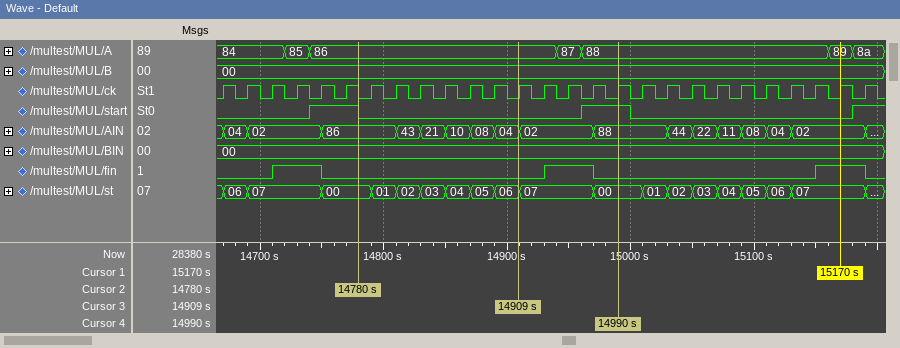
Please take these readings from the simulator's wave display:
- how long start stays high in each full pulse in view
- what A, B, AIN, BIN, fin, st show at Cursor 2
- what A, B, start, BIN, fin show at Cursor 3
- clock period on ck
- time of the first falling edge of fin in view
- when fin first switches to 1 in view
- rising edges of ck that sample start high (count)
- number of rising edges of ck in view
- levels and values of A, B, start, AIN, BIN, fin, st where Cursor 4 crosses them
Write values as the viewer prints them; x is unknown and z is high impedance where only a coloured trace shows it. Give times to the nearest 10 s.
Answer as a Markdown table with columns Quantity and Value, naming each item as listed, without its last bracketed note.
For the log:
| Quantity | Value |
|---|---|
| how long start stays high in each full pulse in view | 40 s, 40 s |
| what A, B, AIN, BIN, fin, st show at Cursor 2 | A=86, B=00, AIN=86, BIN=00, fin=0, st=00 |
| what A, B, start, BIN, fin show at Cursor 3 | A=86, B=00, start=0, BIN=00, fin=0 |
| clock period on ck | 20 s |
| time of the first falling edge of fin in view | 14750 s |
| when fin first switches to 1 in view | 14710 s |
| rising edges of ck that sample start high | 5 |
| number of rising edges of ck in view | 27 |
| levels and values of A, B, start, AIN, BIN, fin, st where Cursor 4 crosses them | A=88, B=00, start=1, AIN=88, BIN=00, fin=0, st=00 |
